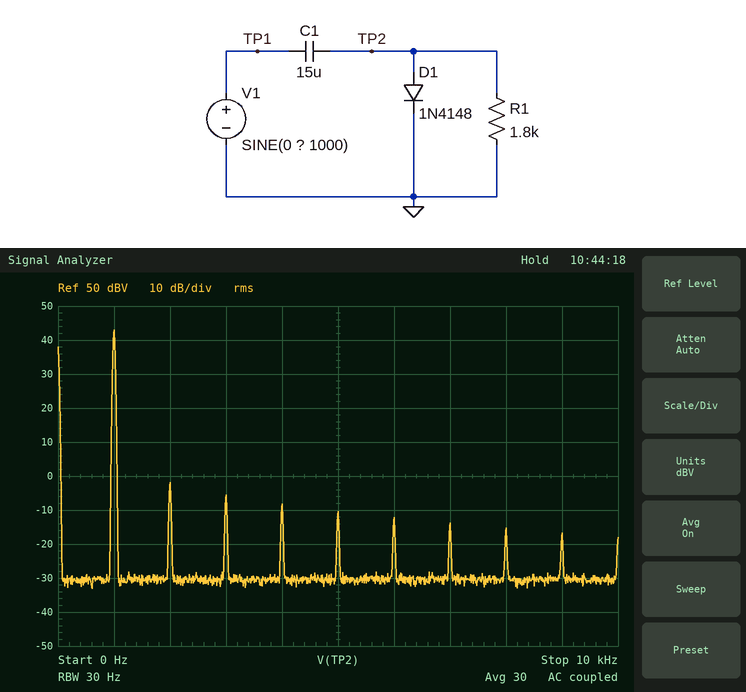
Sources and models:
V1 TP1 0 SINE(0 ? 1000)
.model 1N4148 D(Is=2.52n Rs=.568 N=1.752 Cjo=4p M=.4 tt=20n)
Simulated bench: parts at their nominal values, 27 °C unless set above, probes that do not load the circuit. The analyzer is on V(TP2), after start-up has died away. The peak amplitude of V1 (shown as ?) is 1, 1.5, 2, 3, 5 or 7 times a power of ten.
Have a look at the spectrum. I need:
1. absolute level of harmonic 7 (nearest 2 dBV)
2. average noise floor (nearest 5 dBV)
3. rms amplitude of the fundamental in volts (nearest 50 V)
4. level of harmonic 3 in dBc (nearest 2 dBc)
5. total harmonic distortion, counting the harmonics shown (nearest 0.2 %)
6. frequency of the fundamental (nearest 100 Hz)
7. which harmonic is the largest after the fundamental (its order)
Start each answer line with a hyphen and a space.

- -14 dBV
- -30 dBV
- 150 V
- -48 dBc
- 0.8 %
- 1.0 kHz
- 2
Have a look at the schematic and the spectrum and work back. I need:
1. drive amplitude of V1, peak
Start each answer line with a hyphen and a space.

- 200 V
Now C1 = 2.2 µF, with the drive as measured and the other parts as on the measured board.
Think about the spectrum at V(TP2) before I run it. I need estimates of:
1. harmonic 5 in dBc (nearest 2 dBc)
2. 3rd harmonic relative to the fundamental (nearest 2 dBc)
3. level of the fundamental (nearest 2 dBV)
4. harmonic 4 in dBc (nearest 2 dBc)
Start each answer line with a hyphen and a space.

- -40 dBc
- -34 dBc
- 42 dBV
- -36 dBc
